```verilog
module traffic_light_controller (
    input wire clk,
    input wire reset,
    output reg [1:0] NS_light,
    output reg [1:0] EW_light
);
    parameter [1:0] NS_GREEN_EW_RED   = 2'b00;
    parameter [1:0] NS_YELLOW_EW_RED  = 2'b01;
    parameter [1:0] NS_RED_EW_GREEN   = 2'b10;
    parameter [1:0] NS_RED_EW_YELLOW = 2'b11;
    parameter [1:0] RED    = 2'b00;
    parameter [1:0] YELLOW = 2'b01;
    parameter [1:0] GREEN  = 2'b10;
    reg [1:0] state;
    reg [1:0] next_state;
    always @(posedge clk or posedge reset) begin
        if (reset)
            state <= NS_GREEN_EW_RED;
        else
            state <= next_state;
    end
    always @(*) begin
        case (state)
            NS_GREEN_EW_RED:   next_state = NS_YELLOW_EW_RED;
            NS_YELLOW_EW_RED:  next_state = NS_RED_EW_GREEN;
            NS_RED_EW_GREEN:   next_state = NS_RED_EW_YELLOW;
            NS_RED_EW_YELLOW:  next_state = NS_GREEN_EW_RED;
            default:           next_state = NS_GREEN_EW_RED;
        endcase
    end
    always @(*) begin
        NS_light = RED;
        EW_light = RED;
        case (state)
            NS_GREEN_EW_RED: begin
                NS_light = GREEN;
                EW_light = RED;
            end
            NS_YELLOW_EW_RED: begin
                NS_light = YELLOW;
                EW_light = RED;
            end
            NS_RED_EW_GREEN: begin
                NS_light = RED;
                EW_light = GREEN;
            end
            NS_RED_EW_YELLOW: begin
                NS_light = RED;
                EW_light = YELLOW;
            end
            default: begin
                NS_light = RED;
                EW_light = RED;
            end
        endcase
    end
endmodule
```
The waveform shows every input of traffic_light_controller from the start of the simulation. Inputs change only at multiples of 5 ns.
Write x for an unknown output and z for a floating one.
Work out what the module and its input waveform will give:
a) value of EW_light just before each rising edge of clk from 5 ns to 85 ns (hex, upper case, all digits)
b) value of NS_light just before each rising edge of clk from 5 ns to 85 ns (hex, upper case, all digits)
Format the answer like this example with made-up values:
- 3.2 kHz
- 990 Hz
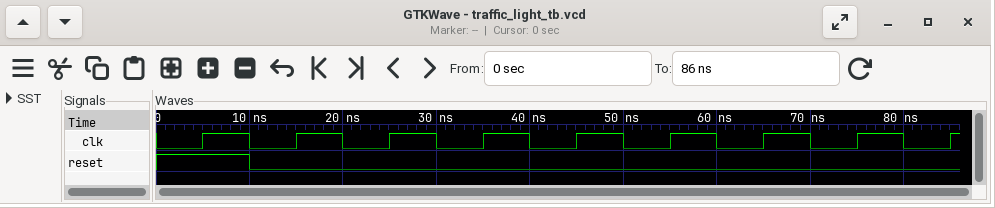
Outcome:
- 0, 0, 0, 2, 1, 0, 0, 2, 1
- 2, 2, 1, 0, 0, 2, 1, 0, 0
